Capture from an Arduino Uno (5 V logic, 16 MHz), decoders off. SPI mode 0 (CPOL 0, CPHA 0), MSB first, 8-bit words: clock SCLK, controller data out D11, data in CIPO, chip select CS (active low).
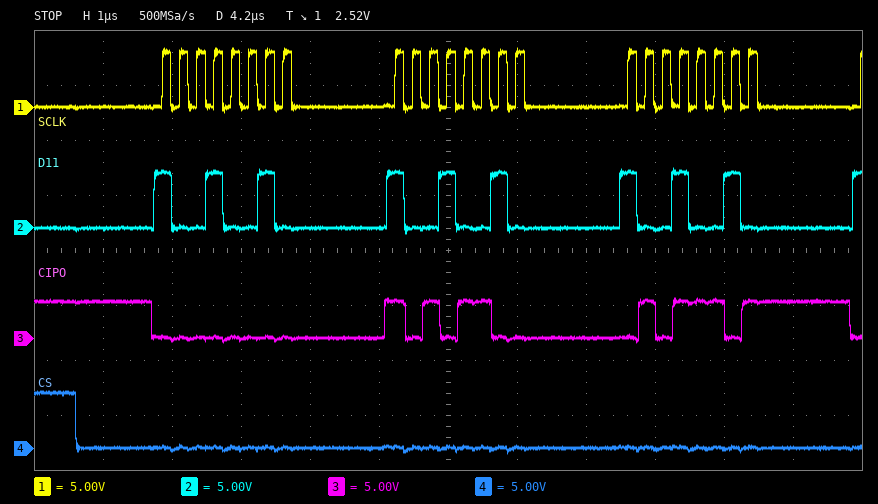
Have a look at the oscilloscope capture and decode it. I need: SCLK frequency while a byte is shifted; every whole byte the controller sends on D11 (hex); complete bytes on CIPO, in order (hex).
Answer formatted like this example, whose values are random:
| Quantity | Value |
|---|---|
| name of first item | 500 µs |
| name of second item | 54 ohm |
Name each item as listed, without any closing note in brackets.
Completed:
| Quantity | Value |
|---|---|
| SCLK frequency while a byte is shifted | 4 MHz |
| every whole byte the controller sends on D11 | 92 92 92 |
| complete bytes on CIPO, in order | 00 AC 5D |
